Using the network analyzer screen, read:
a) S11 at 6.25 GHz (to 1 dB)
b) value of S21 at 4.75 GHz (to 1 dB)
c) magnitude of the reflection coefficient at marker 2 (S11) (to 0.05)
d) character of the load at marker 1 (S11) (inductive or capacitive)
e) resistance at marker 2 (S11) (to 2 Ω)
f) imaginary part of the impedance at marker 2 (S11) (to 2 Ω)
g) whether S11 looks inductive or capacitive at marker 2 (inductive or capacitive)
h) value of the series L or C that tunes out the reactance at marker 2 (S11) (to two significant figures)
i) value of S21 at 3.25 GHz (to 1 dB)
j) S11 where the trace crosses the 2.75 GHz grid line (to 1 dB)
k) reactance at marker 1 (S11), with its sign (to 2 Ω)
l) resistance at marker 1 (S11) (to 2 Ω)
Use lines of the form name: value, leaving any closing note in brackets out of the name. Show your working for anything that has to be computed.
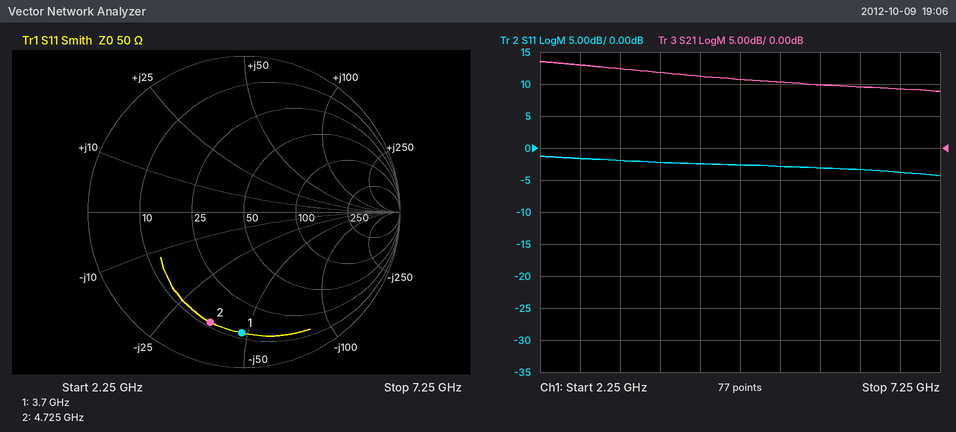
S11 at 6.25 GHz: -3 dB
value of S21 at 4.75 GHz: 11 dB
magnitude of the reflection coefficient at marker 2 (S11): 0.75
character of the load at marker 1 (S11): capacitive
resistance at marker 2 (S11): 12 Ω
imaginary part of the impedance at marker 2 (S11): -36 Ω
whether S11 looks inductive or capacitive at marker 2: capacitive
value of the series L or C that tunes out the reactance at marker 2 (S11): L = 36 Ω/(2π × 4.725 GHz) ≈ 1.2 nH
value of S21 at 3.25 GHz: 12 dB
S11 where the trace crosses the 2.75 GHz grid line: -2 dB
reactance at marker 1 (S11), with its sign: -48 Ω
resistance at marker 1 (S11): 12 Ω
